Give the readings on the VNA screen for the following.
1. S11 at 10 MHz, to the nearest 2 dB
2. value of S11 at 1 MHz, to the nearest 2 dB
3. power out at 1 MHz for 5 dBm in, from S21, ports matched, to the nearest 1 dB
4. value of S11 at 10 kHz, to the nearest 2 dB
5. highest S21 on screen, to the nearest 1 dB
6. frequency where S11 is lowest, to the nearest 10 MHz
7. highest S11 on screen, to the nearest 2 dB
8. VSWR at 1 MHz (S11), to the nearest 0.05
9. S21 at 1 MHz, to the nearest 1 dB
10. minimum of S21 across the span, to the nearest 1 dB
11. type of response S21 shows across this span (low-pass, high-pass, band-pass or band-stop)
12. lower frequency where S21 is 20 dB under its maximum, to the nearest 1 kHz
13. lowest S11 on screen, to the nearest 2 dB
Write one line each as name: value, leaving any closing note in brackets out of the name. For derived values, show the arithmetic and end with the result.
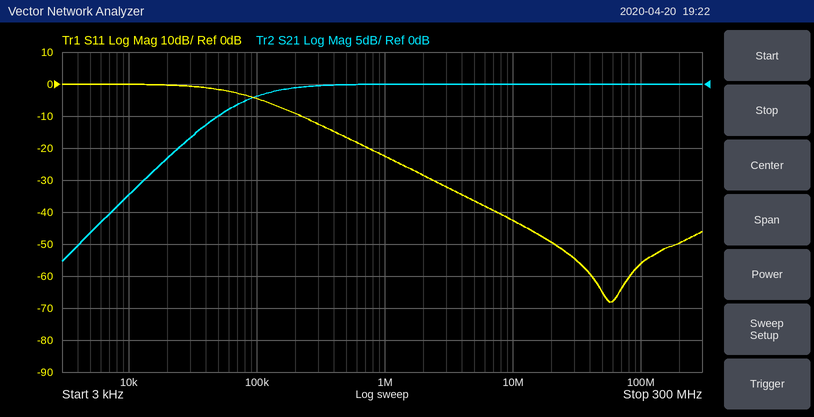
S11 at 10 MHz, to the nearest 2 dB: -42 dB
value of S11 at 1 MHz, to the nearest 2 dB: -22 dB
power out at 1 MHz for 5 dBm in, from S21, ports matched, to the nearest 1 dB: 5 dBm + (0 dB) = 5 dBm
value of S11 at 10 kHz, to the nearest 2 dB: 0 dB
highest S21 on screen, to the nearest 1 dB: 0 dB
frequency where S11 is lowest, to the nearest 10 MHz: 60 MHz
highest S11 on screen, to the nearest 2 dB: 0 dB
VSWR at 1 MHz (S11), to the nearest 0.05: |Γ| = 10^(-22/20) = 0.0794; VSWR = (1 + 0.0794)/(1 − 0.0794) ≈ 1.17, so 1.15 to the nearest 0.05
S21 at 1 MHz, to the nearest 1 dB: 0 dB
minimum of S21 across the span, to the nearest 1 dB: -28 dB
type of response S21 shows across this span: high-pass
lower frequency where S21 is 20 dB under its maximum, to the nearest 1 kHz: 7 kHz
lowest S11 on screen, to the nearest 2 dB: -68 dB
